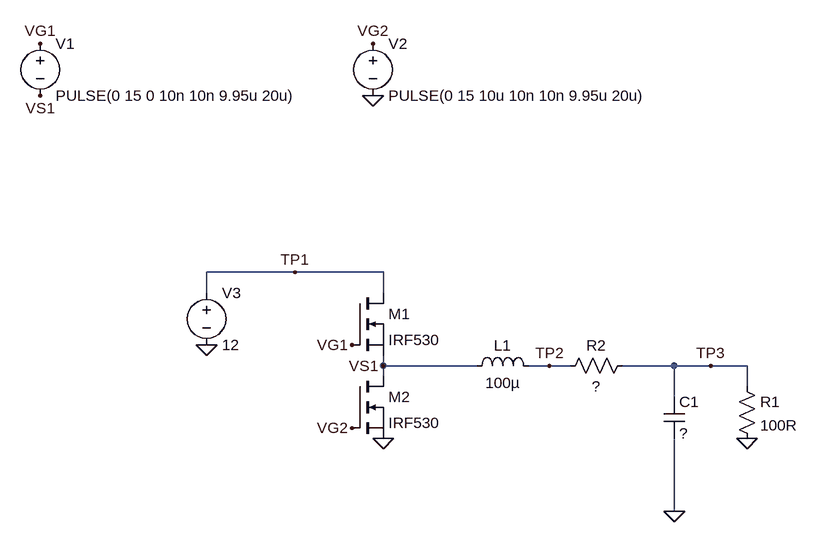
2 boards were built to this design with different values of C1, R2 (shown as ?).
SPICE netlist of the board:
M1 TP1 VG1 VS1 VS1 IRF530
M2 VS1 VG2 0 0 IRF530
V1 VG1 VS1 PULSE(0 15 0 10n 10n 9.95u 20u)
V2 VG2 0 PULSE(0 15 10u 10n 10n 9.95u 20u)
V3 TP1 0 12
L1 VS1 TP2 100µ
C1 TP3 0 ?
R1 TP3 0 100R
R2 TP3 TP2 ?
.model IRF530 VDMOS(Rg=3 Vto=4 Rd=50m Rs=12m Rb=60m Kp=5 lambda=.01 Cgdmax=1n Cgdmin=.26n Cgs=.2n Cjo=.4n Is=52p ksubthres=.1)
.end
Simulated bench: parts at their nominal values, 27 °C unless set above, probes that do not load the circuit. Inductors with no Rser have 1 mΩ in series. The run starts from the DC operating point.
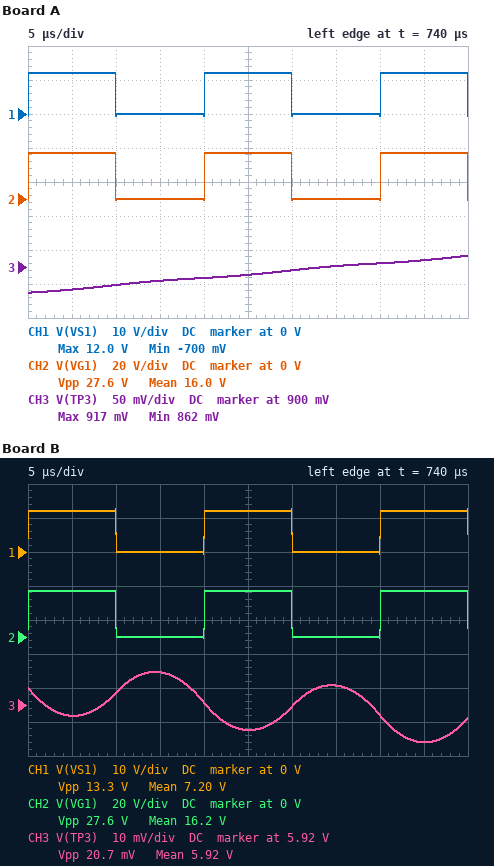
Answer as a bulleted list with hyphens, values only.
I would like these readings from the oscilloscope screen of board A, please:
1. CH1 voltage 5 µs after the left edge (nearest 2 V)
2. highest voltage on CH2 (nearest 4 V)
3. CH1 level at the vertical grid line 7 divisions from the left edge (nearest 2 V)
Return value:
- 12 V
- 28 V
- 0 V
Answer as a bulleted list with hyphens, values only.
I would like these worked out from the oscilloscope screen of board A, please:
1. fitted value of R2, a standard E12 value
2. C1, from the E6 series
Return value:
- 6.8 Ω
- 680 µF
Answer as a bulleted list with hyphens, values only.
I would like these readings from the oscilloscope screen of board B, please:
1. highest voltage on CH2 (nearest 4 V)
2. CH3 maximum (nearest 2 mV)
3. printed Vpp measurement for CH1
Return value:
- 28 V
- 5.930 V
- 13.3 V
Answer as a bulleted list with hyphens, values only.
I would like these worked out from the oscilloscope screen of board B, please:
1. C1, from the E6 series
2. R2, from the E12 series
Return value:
- 100 µF
- 1.5 Ω
